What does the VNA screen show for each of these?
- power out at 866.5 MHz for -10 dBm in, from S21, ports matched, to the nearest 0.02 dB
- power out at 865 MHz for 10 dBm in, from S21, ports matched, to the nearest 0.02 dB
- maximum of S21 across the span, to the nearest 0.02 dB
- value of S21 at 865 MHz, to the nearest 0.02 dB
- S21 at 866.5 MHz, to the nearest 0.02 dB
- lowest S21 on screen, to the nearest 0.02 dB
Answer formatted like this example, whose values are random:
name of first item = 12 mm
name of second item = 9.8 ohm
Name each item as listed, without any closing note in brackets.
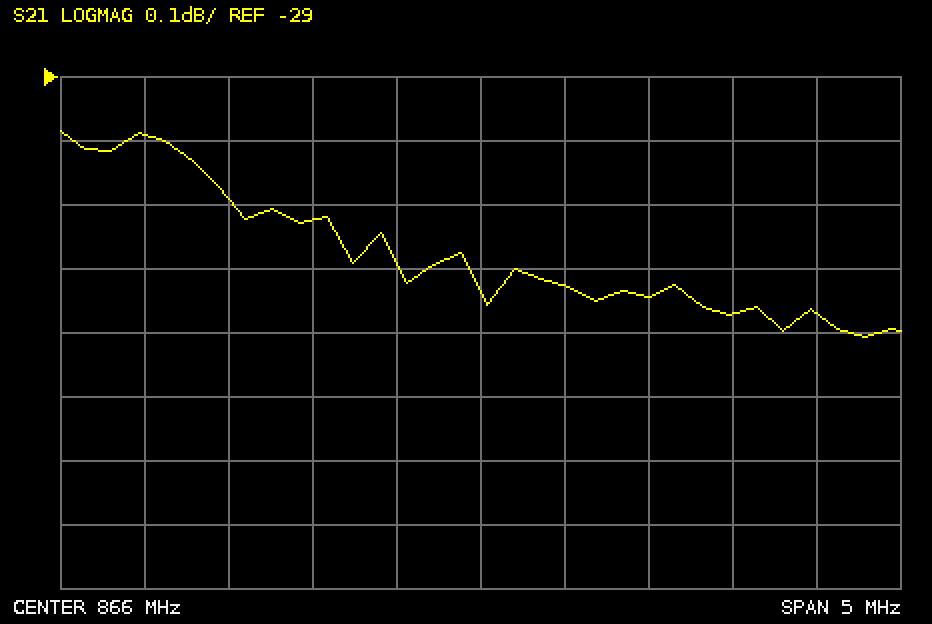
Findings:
power out at 866.5 MHz for -10 dBm in, from S21, ports matched, to the nearest 0.02 dB = -39.32 dBm
power out at 865 MHz for 10 dBm in, from S21, ports matched, to the nearest 0.02 dB = -19.22 dBm
maximum of S21 across the span, to the nearest 0.02 dB = -29.08 dB
value of S21 at 865 MHz, to the nearest 0.02 dB = -29.22 dB
S21 at 866.5 MHz, to the nearest 0.02 dB = -29.32 dB
lowest S21 on screen, to the nearest 0.02 dB = -29.40 dB
